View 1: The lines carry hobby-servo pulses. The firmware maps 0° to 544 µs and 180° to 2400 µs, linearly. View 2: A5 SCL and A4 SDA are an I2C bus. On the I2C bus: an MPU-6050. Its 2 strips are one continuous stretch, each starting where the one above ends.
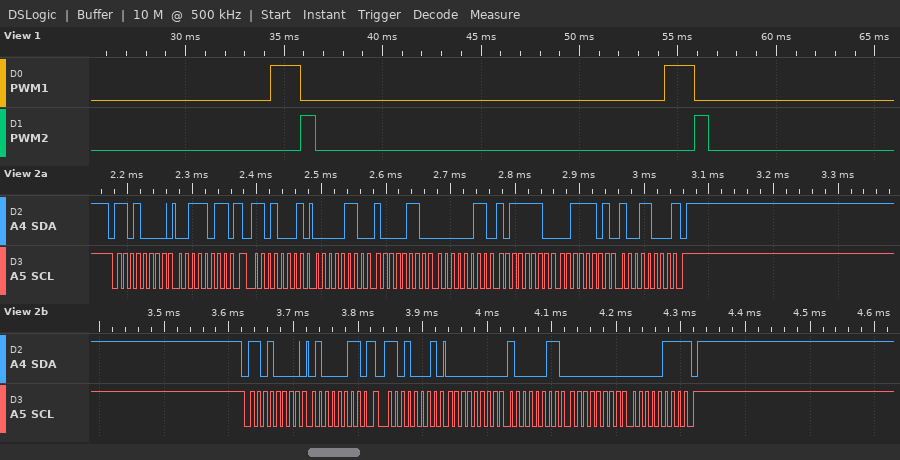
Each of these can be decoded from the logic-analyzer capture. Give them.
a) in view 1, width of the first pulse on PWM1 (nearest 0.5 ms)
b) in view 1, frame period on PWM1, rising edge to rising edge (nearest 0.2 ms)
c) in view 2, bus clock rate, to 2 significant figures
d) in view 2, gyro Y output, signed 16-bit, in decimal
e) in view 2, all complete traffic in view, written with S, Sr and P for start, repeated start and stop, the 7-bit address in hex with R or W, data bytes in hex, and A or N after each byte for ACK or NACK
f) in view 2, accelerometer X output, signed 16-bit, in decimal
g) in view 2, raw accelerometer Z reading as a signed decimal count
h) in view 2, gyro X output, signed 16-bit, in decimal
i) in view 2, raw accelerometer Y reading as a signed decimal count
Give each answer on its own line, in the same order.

1.5 ms
20.0 ms
100 kHz
7
S 68W A 3B A Sr 68R A 06 A 86 A 03 A BE A 3D A 98 N P S 68W A 43 A Sr 68R A 00 A 83 A 00 A 07 N P
1670
15768
131
958
